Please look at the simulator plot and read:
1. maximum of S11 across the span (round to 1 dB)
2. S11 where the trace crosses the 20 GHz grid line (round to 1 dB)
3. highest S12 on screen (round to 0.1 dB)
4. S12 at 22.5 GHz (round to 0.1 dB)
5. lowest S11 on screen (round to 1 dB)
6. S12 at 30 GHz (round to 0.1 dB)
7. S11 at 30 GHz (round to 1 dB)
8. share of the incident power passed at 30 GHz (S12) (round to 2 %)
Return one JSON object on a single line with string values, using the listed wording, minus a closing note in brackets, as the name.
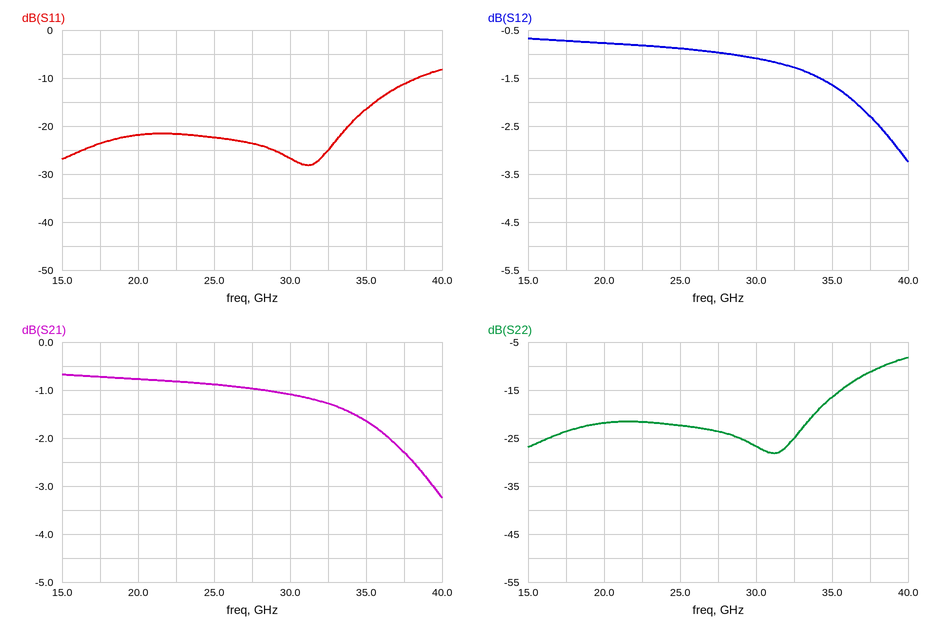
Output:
{"maximum of S11 across the span": "-8 dB", "S11 where the trace crosses the 20 GHz grid line": "-22 dB", "highest S12 on screen": "-0.7 dB", "S12 at 22.5 GHz": "-0.8 dB", "lowest S11 on screen": "-28 dB", "S12 at 30 GHz": "-1.1 dB", "S11 at 30 GHz": "-27 dB", "share of the incident power passed at 30 GHz (S12)": "78 %"}
